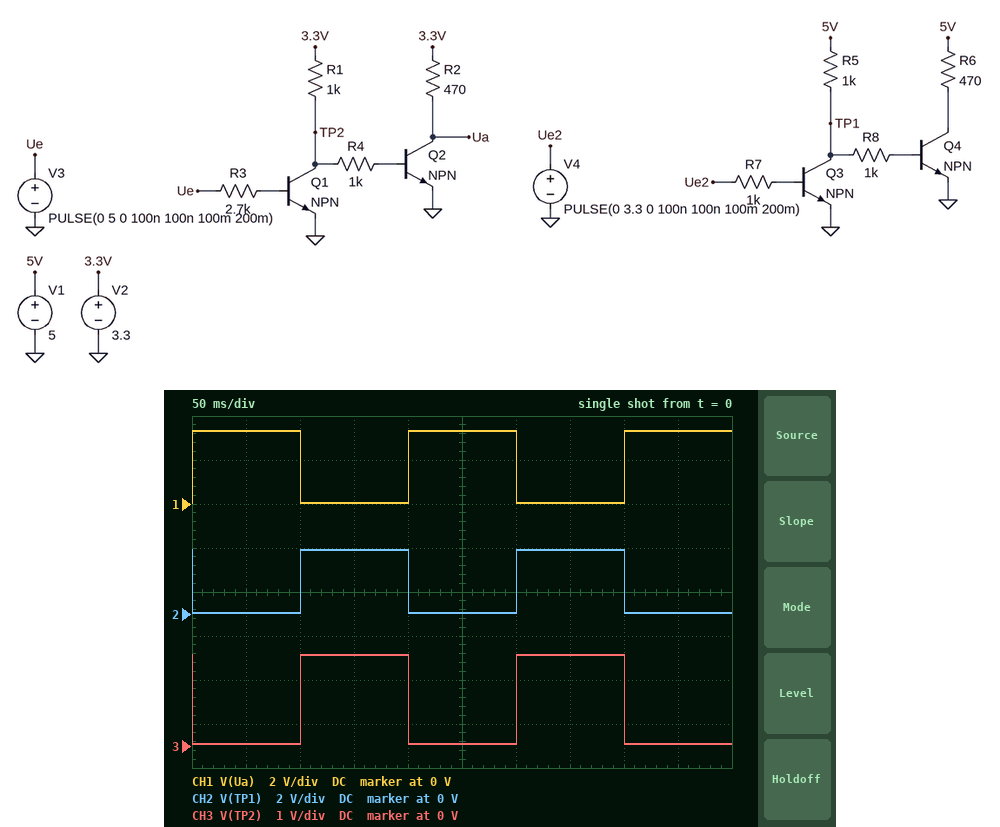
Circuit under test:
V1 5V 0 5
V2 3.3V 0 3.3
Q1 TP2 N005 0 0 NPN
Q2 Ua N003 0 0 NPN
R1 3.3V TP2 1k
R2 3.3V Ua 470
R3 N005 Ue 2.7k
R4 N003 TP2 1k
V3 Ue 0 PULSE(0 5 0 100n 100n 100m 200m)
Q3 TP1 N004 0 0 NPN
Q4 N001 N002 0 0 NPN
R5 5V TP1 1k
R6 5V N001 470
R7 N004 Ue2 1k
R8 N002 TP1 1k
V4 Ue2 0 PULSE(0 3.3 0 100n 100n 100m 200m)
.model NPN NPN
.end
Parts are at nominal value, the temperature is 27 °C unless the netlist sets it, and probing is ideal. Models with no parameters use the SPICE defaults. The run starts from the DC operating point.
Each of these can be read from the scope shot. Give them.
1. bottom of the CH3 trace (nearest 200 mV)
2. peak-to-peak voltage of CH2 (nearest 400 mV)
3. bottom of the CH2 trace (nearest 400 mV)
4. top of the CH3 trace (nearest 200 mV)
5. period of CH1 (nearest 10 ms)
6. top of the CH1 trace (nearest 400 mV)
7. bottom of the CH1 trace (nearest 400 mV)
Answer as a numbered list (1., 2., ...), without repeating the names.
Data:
1. 0 V
2. 2.8 V
3. 0 V
4. 2.0 V
5. 200 ms
6. 3.2 V
7. 0 V
